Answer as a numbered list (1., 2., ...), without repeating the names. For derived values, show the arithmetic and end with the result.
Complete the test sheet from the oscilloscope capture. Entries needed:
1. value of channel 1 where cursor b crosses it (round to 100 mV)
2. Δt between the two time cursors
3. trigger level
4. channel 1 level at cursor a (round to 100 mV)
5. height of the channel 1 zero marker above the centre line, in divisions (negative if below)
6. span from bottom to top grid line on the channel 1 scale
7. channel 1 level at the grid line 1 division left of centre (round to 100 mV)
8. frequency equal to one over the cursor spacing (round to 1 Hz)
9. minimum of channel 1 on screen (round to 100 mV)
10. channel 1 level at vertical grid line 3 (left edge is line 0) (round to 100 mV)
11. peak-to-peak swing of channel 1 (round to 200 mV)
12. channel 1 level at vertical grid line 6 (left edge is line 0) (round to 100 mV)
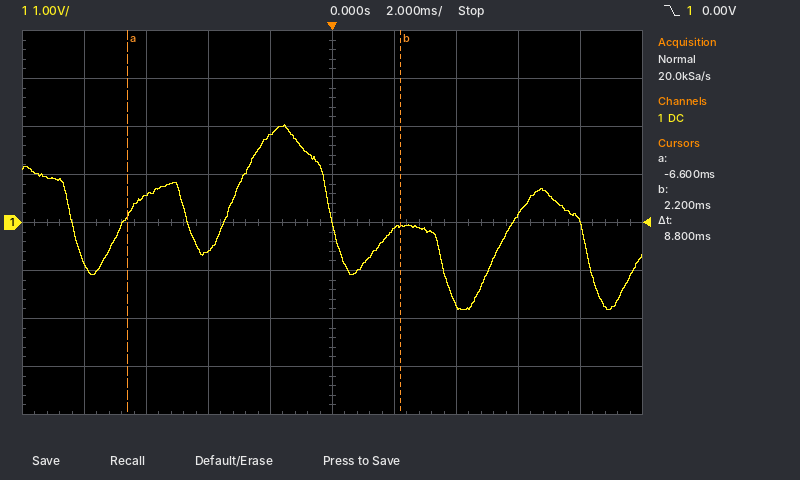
1. -100 mV
2. 8.8 ms
3. 0.00 V
4. 100 mV
5. 0.0 div
6. 8 V
7. 1.8 V
8. 1 / 8.8 ms ≈ 114 Hz
9. -1.8 V
10. -600 mV
11. 3.8 V
12. -100 mV
